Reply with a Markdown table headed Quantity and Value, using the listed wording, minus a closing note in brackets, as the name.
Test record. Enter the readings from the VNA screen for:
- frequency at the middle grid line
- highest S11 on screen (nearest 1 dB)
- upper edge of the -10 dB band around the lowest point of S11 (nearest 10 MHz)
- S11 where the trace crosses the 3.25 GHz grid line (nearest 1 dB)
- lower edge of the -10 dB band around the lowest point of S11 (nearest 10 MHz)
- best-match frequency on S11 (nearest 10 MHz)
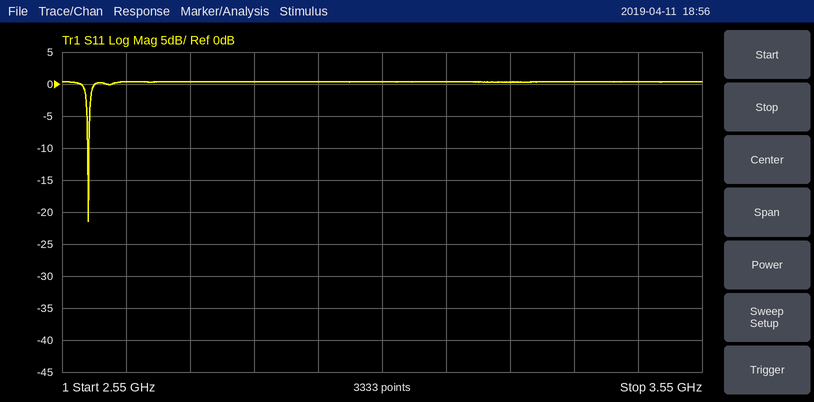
| Quantity | Value |
|---|---|
| frequency at the middle grid line | 3.05 GHz |
| highest S11 on screen | 0 dB |
| upper edge of the -10 dB band around the lowest point of S11 | 2.59 GHz |
| S11 where the trace crosses the 3.25 GHz grid line | 0 dB |
| lower edge of the -10 dB band around the lowest point of S11 | 2.59 GHz |
| best-match frequency on S11 | 2.59 GHz |
